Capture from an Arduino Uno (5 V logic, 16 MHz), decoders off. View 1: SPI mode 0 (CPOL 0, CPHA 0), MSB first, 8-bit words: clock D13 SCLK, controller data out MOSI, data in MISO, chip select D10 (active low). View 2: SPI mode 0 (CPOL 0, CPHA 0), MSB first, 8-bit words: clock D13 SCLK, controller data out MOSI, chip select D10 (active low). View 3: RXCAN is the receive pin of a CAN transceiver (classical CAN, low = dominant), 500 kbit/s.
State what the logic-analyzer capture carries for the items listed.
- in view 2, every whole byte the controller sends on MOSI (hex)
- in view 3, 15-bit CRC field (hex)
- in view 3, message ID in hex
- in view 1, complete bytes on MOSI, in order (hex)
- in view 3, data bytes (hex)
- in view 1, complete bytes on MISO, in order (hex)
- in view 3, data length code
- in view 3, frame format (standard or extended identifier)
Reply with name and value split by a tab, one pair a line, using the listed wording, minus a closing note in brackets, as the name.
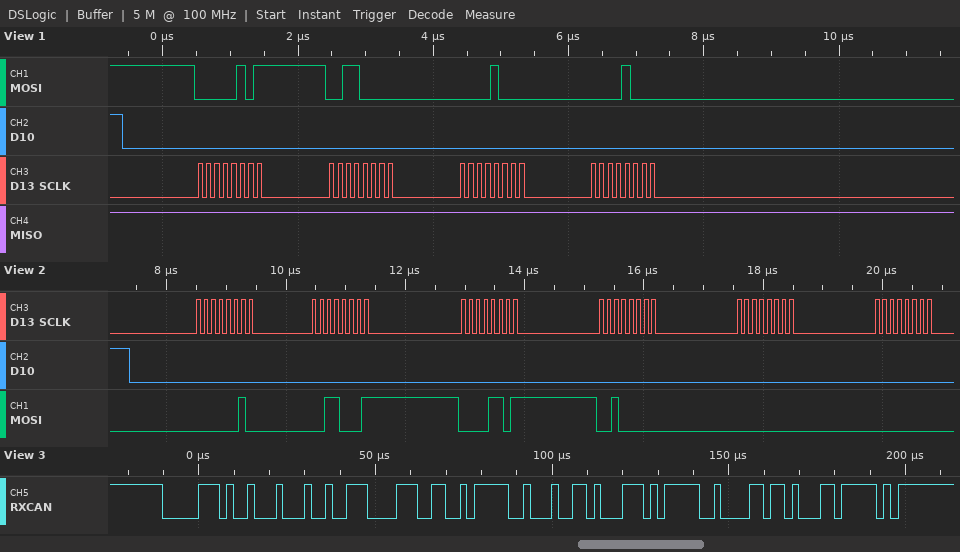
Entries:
in view 2, every whole byte the controller sends on MOSI	02 31 0D 20 00 00
in view 3, 15-bit CRC field	0x68DF
in view 3, message ID in hex	0x069
in view 1, complete bytes on MOSI, in order	0x05 0x30 0x08 0x08
in view 3, data bytes	93 87 32 FA 26 8E BE 86
in view 1, complete bytes on MISO, in order	0xFF 0xFF 0xFF 0xFF
in view 3, data length code	8
in view 3, frame format	standard
